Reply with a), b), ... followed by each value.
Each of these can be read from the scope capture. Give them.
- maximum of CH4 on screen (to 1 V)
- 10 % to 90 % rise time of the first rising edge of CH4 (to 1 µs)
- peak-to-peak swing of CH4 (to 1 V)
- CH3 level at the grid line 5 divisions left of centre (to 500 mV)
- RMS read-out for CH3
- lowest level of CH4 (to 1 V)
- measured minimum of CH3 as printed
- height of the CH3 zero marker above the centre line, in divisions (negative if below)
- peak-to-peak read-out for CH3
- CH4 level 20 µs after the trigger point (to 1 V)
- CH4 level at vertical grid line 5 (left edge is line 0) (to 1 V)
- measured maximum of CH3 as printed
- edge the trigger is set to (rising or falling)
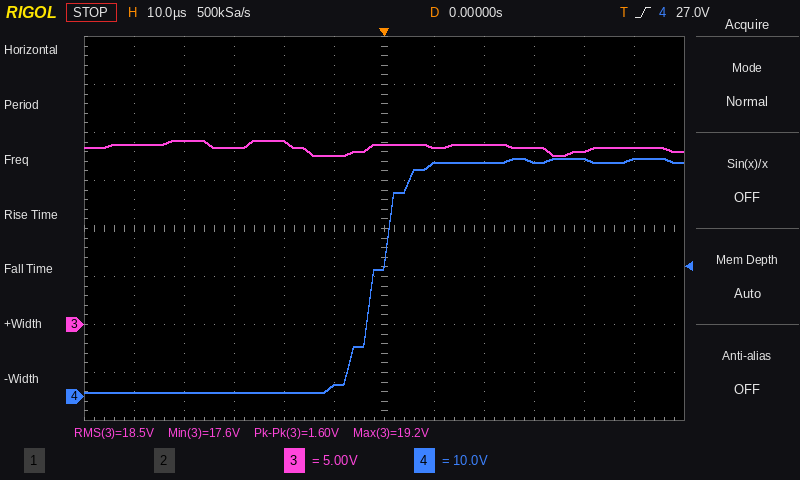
a) 50 V
b) 12 µs
c) 49 V
d) 19.0 V
e) 18.5 V
f) 1 V
g) 17.6 V
h) -2.0 div
i) 1.60 V
j) 49 V
k) 2 V
l) 19.2 V
m) rising
